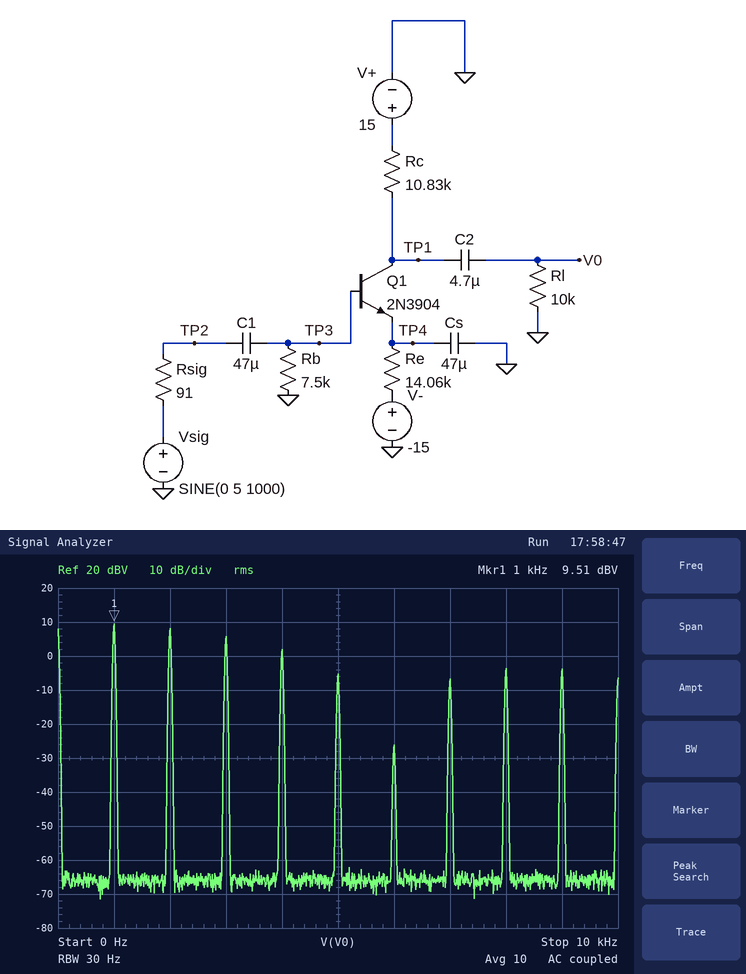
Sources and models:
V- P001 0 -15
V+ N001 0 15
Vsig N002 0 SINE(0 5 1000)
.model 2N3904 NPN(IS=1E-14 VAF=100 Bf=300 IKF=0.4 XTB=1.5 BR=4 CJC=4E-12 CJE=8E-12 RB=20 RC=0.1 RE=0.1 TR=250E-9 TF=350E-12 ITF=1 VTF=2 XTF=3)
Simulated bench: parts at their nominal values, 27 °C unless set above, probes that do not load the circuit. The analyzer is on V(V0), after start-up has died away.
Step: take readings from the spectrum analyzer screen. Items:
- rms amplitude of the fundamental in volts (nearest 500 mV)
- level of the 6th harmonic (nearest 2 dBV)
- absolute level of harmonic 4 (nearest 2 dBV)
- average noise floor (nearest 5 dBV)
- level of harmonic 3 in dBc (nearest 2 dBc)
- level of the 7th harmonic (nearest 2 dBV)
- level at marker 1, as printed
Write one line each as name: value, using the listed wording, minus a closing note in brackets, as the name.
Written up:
rms amplitude of the fundamental in volts: 3.0 V
level of the 6th harmonic: -26 dBV
absolute level of harmonic 4: 2 dBV
average noise floor: -65 dBV
level of harmonic 3 in dBc: -4 dBc
level of the 7th harmonic: -6 dBV
level at marker 1, as printed: 9.51 dBV
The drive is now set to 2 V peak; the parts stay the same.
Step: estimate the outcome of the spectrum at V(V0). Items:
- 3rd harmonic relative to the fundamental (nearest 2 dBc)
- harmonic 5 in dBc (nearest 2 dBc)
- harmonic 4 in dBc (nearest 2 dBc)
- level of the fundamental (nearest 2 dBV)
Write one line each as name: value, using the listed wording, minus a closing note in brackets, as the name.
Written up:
3rd harmonic relative to the fundamental: -6 dBc
harmonic 5 in dBc: -30 dBc
harmonic 4 in dBc: -14 dBc
level of the fundamental: 12 dBV
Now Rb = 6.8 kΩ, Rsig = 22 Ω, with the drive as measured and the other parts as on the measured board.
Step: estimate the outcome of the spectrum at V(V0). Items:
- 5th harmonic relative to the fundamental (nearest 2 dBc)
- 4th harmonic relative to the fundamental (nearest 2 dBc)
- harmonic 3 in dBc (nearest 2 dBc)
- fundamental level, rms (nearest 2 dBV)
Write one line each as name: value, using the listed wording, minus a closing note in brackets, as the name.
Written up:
5th harmonic relative to the fundamental: -8 dBc
4th harmonic relative to the fundamental: -4 dBc
harmonic 3 in dBc: -2 dBc
fundamental level, rms: 8 dBV
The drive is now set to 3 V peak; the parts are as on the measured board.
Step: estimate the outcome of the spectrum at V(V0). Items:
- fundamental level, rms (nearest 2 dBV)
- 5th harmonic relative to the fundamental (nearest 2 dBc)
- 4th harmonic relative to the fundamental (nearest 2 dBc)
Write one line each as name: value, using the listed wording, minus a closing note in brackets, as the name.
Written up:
fundamental level, rms: 10 dBV
5th harmonic relative to the fundamental: -24 dBc
4th harmonic relative to the fundamental: -10 dBc
